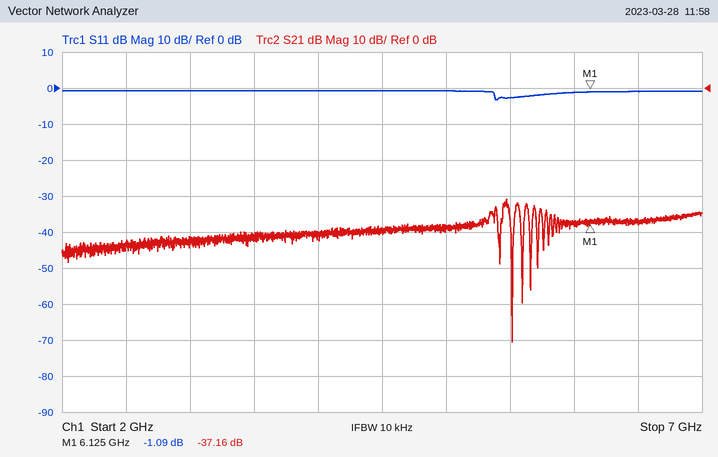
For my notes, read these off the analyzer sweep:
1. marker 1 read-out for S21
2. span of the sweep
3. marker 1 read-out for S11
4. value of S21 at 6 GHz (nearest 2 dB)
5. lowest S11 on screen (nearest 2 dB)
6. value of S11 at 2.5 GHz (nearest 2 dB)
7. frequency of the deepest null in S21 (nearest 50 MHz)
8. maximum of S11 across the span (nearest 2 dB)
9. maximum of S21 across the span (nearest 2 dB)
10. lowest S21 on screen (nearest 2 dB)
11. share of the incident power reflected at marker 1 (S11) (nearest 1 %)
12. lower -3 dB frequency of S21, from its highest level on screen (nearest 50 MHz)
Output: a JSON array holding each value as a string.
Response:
["-37.16 dB", "5 GHz", "-1.09 dB", "-38 dB", "-4 dB", "0 dB", "5.50 GHz", "0 dB", "-30 dB", "-70 dB", "78 %", "5.45 GHz"]
